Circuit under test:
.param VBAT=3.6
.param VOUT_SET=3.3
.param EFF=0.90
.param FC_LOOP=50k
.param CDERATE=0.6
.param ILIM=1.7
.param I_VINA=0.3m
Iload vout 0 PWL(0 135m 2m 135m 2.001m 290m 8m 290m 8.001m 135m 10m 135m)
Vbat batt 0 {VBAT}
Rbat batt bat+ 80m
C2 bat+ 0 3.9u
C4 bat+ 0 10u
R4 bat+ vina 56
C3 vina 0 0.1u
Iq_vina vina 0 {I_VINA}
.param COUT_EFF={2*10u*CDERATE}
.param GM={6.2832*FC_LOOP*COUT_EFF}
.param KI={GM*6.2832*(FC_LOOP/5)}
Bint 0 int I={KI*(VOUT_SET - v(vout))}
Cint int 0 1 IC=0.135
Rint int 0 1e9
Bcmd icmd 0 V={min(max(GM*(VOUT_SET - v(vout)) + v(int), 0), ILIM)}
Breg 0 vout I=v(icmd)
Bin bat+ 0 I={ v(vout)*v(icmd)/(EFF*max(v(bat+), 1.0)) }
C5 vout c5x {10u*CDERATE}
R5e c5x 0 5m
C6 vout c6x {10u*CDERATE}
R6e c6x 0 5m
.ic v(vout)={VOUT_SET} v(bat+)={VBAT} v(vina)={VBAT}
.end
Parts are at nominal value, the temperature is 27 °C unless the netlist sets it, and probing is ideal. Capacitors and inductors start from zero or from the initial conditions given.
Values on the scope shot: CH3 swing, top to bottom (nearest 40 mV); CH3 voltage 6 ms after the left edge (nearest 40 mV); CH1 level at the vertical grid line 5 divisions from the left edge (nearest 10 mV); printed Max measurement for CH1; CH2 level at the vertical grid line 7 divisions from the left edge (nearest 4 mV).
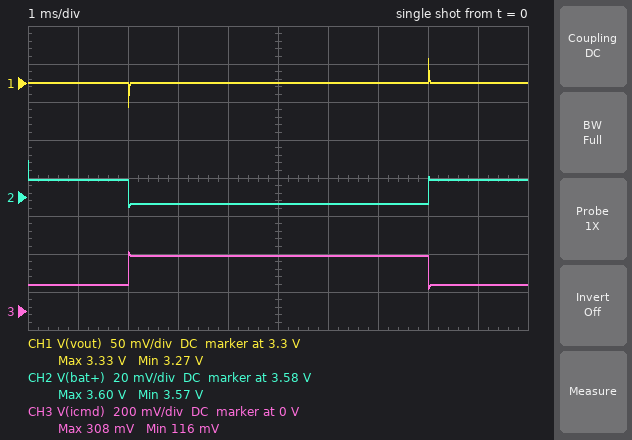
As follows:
200 mV
280 mV
3.30 V
3.33 V
3.576 V
